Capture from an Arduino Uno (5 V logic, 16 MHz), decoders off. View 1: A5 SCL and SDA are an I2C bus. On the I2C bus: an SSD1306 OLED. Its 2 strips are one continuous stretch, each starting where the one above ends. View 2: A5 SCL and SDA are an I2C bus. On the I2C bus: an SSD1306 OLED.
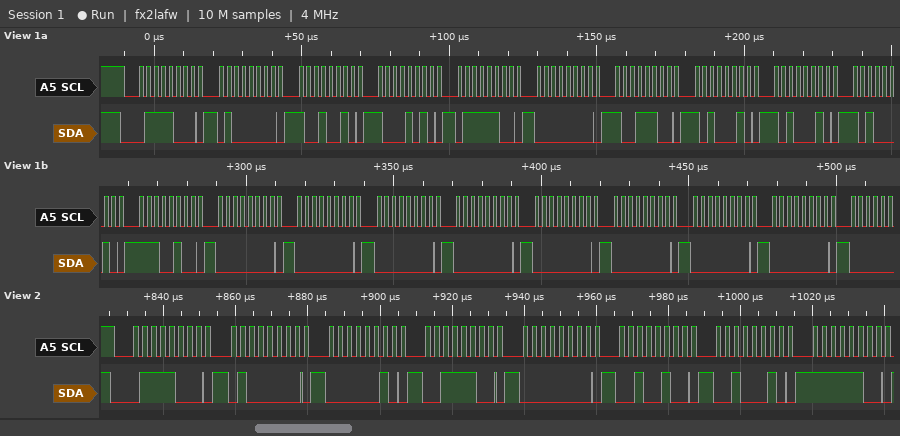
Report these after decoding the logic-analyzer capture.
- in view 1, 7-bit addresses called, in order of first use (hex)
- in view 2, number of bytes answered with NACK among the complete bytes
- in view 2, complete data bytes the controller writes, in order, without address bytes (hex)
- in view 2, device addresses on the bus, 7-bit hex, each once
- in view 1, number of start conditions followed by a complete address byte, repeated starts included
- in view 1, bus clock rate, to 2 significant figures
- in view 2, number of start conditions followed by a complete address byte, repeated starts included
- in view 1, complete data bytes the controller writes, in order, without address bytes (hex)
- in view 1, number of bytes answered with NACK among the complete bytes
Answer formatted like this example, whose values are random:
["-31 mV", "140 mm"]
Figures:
["0x3C", "0", "40 02 3C 00 24 22 FC", "0x3C", "1", "400 kHz", "1", "40 92 8A 7C 00 9C A2 A2 A2 E4 00 00 00 00 00 00 00 00", "0"]
